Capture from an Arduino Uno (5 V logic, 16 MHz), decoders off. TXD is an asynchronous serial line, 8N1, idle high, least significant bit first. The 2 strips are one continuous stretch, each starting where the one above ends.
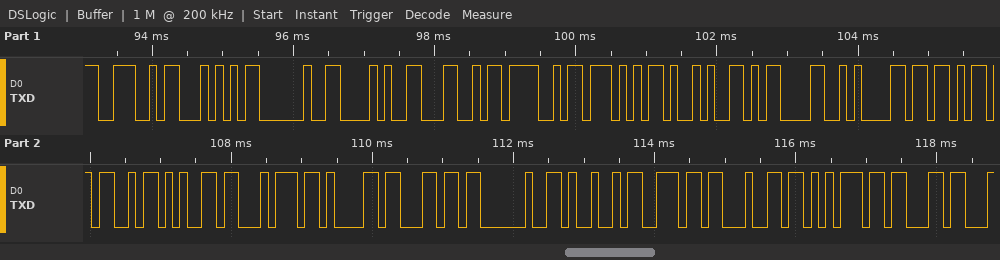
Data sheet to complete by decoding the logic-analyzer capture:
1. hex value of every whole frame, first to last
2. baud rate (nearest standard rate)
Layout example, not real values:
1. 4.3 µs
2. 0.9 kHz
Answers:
1. 4E 54 20 28 4C 4F 57 29 0D 0A 5B 4D 65 74 61 6C 20 49 6E 64 75 63
2. 9600 baud
